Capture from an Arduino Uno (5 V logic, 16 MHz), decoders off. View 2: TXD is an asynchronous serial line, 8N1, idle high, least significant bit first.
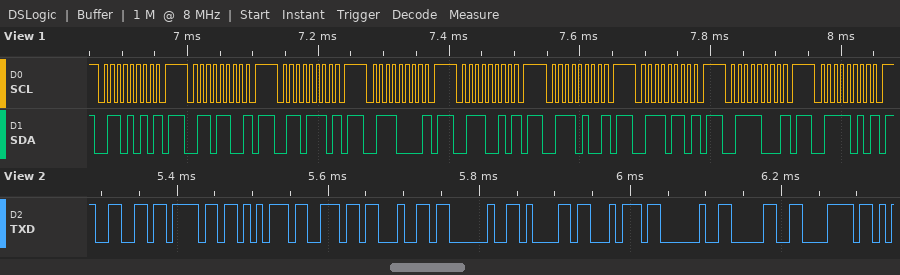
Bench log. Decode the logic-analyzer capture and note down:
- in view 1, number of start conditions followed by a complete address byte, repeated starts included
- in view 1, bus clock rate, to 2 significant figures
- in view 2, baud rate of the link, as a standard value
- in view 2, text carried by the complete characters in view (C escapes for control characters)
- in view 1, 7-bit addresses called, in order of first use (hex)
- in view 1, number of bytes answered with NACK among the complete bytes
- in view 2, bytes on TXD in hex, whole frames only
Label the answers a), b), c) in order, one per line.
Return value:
a) 9
b) 100 kHz
c) 115200 baud
d) "found at 0x"
e) 0x35 0x36 0x37 0x38 0x39 0x3A 0x3B 0x3C 0x3D
f) 9
g) 66 6F 75 6E 64 20 61 74 20 30 78
